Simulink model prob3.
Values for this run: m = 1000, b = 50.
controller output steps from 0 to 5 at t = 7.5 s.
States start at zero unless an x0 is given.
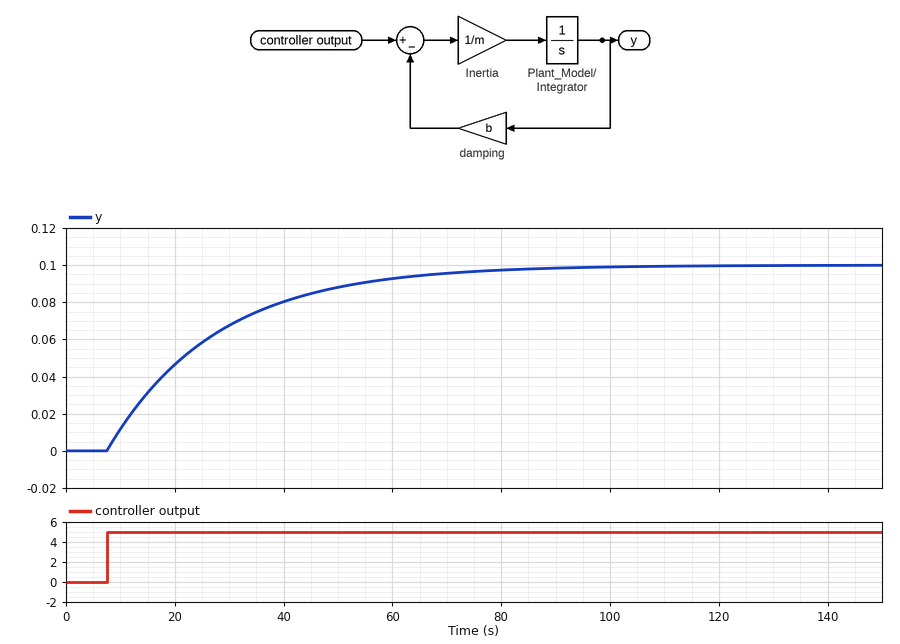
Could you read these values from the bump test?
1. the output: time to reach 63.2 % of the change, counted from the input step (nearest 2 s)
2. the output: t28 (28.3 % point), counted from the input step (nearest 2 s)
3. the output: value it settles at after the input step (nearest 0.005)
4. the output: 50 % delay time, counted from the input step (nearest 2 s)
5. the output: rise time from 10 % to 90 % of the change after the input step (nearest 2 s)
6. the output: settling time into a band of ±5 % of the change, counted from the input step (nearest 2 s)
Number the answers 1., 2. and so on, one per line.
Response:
1. 20 s
2. 6 s
3. 0.100
4. 14 s
5. 44 s
6. 60 s
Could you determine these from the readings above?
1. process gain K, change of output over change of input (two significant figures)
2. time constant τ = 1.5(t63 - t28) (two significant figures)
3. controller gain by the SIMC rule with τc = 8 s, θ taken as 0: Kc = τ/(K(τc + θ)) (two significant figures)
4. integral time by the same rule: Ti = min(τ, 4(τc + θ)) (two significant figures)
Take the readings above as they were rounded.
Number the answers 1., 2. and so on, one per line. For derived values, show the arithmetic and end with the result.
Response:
1. (0.1 - 0) / 5 = 0.020
2. 1.5 × (20 - 6) = 21 s
3. 21 / (0.02 × (8 + 0)) = 130
4. min(21, 4 × (8 + 0)) = 21 s
